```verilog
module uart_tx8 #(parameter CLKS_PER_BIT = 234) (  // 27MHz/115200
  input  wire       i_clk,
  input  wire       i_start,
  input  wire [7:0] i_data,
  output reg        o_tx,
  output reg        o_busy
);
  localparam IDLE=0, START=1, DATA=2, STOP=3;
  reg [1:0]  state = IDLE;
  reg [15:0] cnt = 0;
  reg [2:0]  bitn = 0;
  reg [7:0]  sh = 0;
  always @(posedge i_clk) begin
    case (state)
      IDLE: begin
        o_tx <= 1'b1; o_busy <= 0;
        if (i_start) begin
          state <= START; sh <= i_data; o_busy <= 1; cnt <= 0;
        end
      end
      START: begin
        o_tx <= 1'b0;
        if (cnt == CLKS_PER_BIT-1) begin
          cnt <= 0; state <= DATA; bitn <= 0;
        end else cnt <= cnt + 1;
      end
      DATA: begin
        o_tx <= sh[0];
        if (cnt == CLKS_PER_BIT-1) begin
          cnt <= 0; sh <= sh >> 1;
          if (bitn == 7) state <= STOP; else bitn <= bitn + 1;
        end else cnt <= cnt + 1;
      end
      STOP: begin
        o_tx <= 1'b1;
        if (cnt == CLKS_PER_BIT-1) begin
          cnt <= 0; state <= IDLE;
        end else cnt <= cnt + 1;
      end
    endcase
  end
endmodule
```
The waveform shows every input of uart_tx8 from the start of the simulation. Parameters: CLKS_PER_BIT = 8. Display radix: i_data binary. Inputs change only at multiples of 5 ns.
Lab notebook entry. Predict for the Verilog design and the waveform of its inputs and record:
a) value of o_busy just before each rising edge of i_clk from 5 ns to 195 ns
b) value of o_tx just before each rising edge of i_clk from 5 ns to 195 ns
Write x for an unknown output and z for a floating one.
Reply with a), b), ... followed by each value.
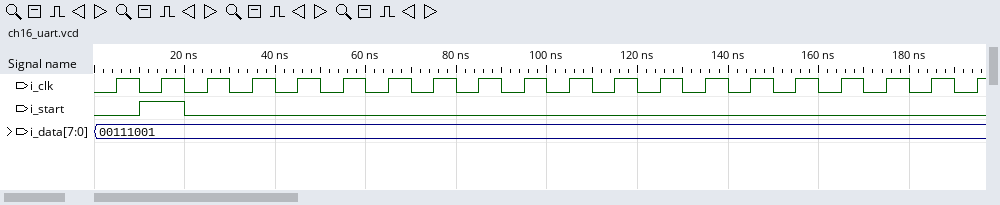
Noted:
a) x 0 1 1 1 1 1 1 1 1 1 1 1 1 1 1 1 1 1 1
b) x 1 1 0 0 0 0 0 0 0 0 1 1 1 1 1 1 1 1 0
